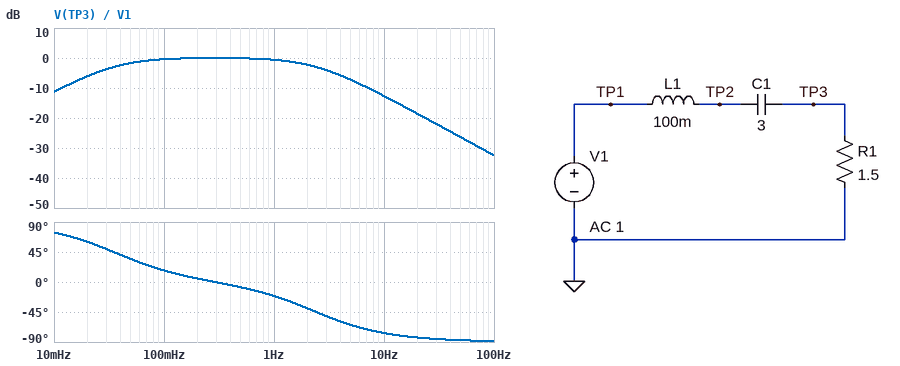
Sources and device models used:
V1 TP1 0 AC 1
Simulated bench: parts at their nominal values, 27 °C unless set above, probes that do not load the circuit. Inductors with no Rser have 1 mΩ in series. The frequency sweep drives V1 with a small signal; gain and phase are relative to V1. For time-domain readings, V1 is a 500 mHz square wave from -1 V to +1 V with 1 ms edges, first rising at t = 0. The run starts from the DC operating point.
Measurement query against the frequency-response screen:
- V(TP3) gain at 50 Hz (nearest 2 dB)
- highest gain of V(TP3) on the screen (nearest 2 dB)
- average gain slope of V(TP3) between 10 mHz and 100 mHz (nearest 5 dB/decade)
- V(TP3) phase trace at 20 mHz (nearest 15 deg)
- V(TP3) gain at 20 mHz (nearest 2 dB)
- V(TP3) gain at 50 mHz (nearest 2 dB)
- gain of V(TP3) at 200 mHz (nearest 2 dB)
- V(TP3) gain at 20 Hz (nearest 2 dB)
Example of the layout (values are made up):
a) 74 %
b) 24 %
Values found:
a) -26 dB
b) 0 dB
c) 10 dB/decade
d) 60 deg
e) -6 dB
f) -2 dB
g) 0 dB
h) -18 dB
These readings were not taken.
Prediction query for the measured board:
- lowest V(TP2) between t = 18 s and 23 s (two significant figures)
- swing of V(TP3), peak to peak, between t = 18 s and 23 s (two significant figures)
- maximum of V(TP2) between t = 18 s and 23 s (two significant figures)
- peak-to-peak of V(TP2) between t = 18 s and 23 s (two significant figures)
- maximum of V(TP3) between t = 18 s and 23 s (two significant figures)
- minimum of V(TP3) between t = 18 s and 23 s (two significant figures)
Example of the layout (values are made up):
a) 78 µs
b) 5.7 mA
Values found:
a) -1.0 V
b) 2.1 V
c) 1.0 V
d) 2.0 V
e) 1.1 V
f) -1.0 V
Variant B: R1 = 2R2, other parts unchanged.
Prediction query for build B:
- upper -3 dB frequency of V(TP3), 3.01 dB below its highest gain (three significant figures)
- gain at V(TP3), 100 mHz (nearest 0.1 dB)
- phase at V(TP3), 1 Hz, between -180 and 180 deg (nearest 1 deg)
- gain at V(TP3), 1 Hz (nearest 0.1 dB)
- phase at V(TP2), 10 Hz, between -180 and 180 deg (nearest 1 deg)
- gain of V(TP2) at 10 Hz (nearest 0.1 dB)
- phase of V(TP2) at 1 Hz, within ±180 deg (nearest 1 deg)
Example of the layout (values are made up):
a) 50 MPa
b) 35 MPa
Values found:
a) 3.53 Hz
b) -0.2 dB
c) -15 deg
d) -0.3 dB
e) -71 deg
f) -9.6 dB
g) -16 deg
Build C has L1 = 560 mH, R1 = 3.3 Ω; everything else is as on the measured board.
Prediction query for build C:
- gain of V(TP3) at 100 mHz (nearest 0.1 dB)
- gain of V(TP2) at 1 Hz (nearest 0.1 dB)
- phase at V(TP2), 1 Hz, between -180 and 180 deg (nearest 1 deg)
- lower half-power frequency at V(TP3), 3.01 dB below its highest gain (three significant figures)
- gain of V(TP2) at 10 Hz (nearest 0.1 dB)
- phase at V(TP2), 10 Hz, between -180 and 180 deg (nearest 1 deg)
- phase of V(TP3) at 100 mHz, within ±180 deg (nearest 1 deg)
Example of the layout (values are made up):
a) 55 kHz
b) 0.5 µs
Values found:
a) 0 dB
b) -3.2 dB
c) -47 deg
d) 15.8 mHz
e) -20.6 dB
f) -85 deg
g) 3 deg
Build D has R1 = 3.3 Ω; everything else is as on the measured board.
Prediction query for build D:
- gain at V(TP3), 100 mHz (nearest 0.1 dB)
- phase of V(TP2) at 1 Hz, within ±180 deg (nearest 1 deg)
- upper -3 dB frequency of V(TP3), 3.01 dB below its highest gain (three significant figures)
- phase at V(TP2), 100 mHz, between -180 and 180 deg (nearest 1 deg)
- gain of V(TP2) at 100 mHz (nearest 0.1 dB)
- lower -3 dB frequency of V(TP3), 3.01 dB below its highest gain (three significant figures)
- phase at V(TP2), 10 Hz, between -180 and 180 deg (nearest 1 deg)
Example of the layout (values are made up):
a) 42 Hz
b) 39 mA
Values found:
a) -0.1 dB
b) -11 deg
c) 5.27 Hz
d) -1 deg
e) 0 dB
f) 16.0 mHz
g) -62 deg
